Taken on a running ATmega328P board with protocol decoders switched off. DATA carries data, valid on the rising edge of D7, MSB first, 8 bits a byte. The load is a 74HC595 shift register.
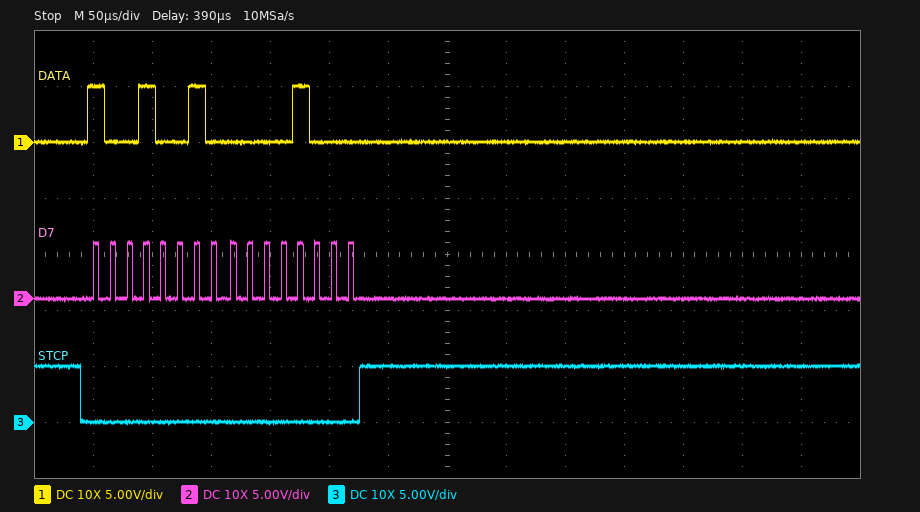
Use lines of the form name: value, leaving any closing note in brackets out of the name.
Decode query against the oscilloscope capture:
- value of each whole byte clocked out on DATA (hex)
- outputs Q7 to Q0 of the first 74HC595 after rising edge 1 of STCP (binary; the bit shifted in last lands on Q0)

value of each whole byte clocked out on DATA: 92 08
outputs Q7 to Q0 of the first 74HC595 after rising edge 1 of STCP: 00001000
